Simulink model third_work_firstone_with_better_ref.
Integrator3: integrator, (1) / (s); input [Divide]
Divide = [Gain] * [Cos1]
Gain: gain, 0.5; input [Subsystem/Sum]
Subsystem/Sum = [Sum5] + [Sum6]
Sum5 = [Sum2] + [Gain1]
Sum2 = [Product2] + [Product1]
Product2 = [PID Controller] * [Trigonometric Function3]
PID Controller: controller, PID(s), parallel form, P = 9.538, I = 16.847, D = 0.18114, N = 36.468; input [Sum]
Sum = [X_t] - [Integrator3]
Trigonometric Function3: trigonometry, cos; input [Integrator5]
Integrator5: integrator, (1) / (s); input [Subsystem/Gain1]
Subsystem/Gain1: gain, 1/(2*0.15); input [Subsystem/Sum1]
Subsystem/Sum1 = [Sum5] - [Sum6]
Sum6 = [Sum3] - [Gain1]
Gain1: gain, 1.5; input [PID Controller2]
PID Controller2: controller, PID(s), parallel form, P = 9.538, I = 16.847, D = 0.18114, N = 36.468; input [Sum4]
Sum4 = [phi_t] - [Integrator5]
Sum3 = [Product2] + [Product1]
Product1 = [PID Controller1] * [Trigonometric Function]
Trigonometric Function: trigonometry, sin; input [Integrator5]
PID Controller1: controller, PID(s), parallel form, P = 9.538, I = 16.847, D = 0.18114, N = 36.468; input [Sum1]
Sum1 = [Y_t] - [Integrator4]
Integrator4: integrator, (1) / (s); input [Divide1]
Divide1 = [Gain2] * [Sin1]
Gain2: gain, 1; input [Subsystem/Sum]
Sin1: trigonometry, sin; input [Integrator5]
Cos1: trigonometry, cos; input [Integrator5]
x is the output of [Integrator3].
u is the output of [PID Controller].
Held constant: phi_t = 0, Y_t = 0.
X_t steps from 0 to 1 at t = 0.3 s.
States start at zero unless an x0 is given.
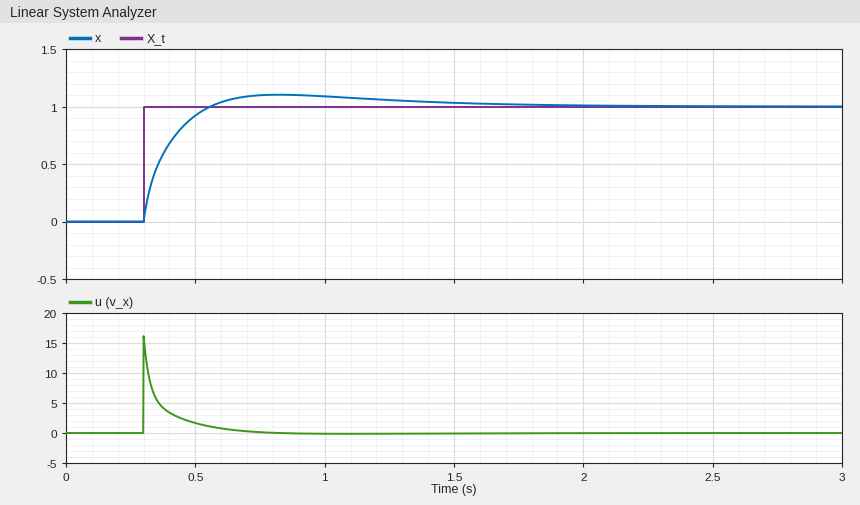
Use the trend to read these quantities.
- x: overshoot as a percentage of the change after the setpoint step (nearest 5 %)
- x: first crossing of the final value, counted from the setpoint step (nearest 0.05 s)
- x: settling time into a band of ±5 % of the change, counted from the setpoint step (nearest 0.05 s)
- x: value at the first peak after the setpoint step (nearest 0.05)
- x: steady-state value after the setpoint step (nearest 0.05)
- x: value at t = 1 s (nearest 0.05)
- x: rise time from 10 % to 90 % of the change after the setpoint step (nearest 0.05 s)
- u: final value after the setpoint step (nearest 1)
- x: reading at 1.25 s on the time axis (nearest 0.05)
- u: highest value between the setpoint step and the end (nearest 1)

10 %
0.25 s
1.00 s
1.10
1.00
1.10
0.20 s
0
1.05
16
